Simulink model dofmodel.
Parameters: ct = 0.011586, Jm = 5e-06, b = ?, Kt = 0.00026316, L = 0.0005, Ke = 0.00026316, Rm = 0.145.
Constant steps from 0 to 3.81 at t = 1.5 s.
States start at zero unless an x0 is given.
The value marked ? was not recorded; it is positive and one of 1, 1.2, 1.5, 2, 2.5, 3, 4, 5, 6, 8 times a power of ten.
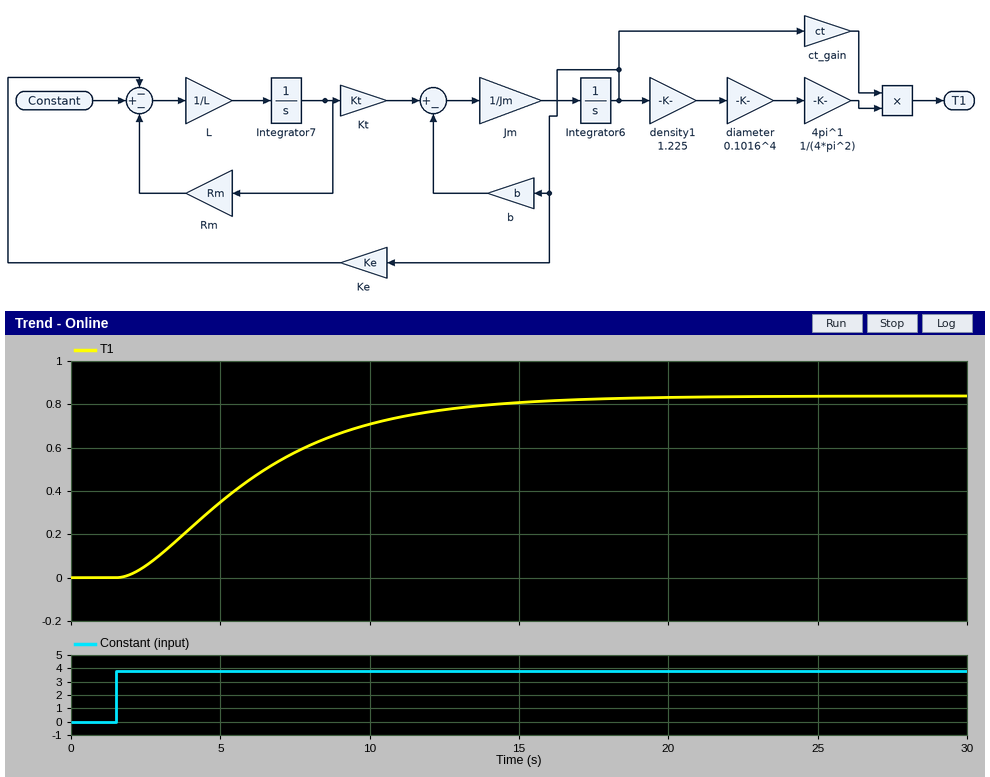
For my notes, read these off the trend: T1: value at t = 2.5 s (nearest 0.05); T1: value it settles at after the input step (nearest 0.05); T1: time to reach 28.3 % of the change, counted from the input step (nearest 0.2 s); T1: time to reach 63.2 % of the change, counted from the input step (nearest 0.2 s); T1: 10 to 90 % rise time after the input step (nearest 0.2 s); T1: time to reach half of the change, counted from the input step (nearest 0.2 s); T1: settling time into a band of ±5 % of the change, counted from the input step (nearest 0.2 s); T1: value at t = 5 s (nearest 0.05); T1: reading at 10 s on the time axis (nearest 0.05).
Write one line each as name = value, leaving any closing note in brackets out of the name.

T1: value at t = 2.5 s = 0.05
T1: value it settles at after the input step = 0.85
T1: time to reach 28.3 % of the change, counted from the input step = 2.6 s
T1: time to reach 63.2 % of the change, counted from the input step = 5.4 s
T1: 10 to 90 % rise time after the input step = 8.8 s
T1: time to reach half of the change, counted from the input step = 4.2 s
T1: settling time into a band of ±5 % of the change, counted from the input step = 12.4 s
T1: value at t = 5 s = 0.35
T1: reading at 10 s on the time axis = 0.70
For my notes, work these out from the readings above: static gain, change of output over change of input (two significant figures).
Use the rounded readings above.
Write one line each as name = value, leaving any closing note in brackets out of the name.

static gain, change of output over change of input = 0.22
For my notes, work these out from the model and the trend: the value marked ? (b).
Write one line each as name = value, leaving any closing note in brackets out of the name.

the value marked ? = 1e-06
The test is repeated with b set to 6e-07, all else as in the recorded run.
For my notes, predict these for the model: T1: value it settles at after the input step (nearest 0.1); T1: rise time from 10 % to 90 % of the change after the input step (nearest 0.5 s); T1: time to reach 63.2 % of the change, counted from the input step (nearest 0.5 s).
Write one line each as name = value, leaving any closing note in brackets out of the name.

T1: value it settles at after the input step = 1.6
T1: rise time from 10 % to 90 % of the change after the input step = 12.0 s
T1: time to reach 63.2 % of the change, counted from the input step = 7.5 s
